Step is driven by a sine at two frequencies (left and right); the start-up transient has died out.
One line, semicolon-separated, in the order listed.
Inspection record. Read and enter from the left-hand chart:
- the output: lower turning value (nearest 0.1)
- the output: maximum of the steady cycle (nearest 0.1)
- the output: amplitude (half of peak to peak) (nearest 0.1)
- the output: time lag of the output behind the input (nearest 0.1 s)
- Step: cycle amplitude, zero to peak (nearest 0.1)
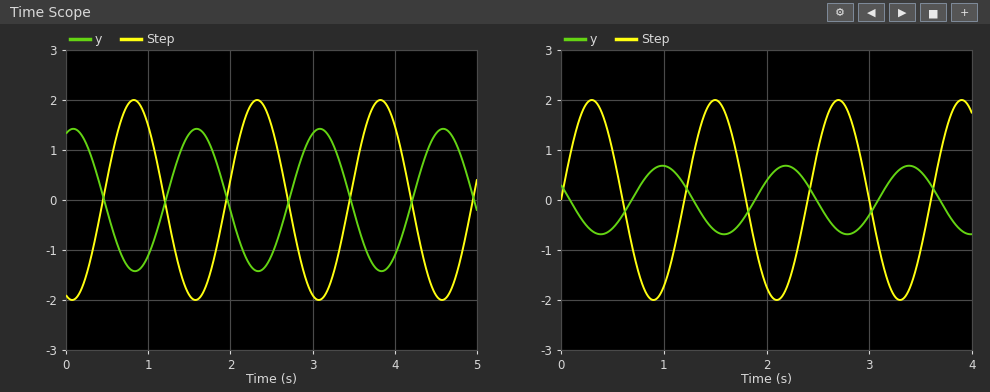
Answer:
-1.4; 1.4; 1.4; 0.8 s; 2.0
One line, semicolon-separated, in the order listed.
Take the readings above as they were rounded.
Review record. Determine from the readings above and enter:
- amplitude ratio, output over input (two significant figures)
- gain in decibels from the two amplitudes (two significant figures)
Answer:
0.70; -3.1 dB
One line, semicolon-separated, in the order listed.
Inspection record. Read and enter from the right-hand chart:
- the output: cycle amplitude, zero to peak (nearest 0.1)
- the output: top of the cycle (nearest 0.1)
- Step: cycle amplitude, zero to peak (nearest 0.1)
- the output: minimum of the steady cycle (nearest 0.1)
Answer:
0.7; 0.7; 2.0; -0.7
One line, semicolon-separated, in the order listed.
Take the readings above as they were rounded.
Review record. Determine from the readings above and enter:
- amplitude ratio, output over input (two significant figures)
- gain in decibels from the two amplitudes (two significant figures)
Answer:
0.35; -9.1 dB
